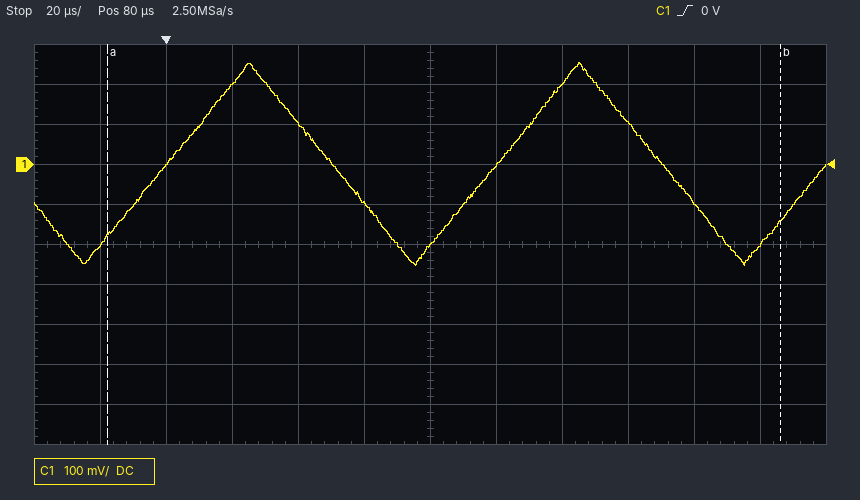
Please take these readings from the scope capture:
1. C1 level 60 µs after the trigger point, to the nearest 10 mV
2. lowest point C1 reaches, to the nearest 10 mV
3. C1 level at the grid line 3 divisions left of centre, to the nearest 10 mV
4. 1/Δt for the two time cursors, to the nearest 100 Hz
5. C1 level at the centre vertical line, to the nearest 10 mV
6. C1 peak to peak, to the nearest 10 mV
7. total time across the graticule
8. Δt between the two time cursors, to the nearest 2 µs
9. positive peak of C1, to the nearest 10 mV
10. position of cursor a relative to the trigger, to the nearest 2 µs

-100 mV
-250 mV
200 mV
4.9 kHz
-200 mV
510 mV
240 µs
204 µs
260 mV
-18 µs
